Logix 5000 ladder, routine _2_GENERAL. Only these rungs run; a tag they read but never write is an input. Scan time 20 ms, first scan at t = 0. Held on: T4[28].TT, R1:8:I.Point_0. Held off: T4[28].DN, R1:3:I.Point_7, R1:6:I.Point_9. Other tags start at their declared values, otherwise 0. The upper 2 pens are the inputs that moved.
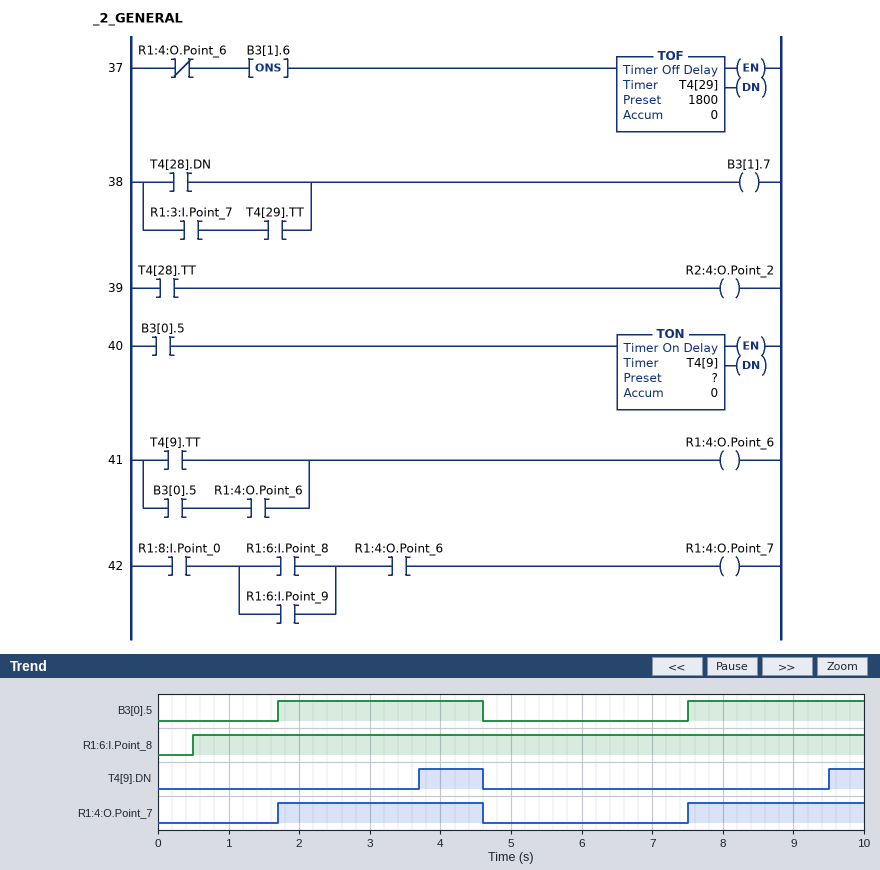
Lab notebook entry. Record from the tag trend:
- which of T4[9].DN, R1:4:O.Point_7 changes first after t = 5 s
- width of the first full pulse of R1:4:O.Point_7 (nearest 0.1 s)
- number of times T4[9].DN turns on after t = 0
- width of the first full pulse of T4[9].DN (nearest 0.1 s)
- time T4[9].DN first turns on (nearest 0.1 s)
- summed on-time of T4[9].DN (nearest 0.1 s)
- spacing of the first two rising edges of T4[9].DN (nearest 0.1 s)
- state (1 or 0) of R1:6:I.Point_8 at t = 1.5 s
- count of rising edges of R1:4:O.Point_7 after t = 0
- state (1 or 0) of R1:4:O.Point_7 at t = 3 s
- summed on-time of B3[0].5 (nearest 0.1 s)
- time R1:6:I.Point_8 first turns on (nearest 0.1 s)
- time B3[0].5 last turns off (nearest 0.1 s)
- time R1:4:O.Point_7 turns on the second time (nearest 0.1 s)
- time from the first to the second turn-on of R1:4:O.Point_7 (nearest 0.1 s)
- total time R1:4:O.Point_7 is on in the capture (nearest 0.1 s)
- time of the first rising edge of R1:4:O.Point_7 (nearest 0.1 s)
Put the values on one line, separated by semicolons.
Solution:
R1:4:O.Point_7; 2.9 s; 2; 0.9 s; 3.7 s; 1.4 s; 5.8 s; 1; 2; 1; 5.4 s; 0.5 s; 4.6 s; 7.5 s; 5.8 s; 5.4 s; 1.7 s
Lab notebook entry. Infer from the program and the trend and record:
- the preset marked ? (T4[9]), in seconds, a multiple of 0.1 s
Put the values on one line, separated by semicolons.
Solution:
2.0 s
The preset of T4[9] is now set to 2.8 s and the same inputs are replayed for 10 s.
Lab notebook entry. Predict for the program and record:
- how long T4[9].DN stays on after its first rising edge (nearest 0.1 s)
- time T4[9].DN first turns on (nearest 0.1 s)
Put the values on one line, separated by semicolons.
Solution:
0.1 s; 4.5 s
